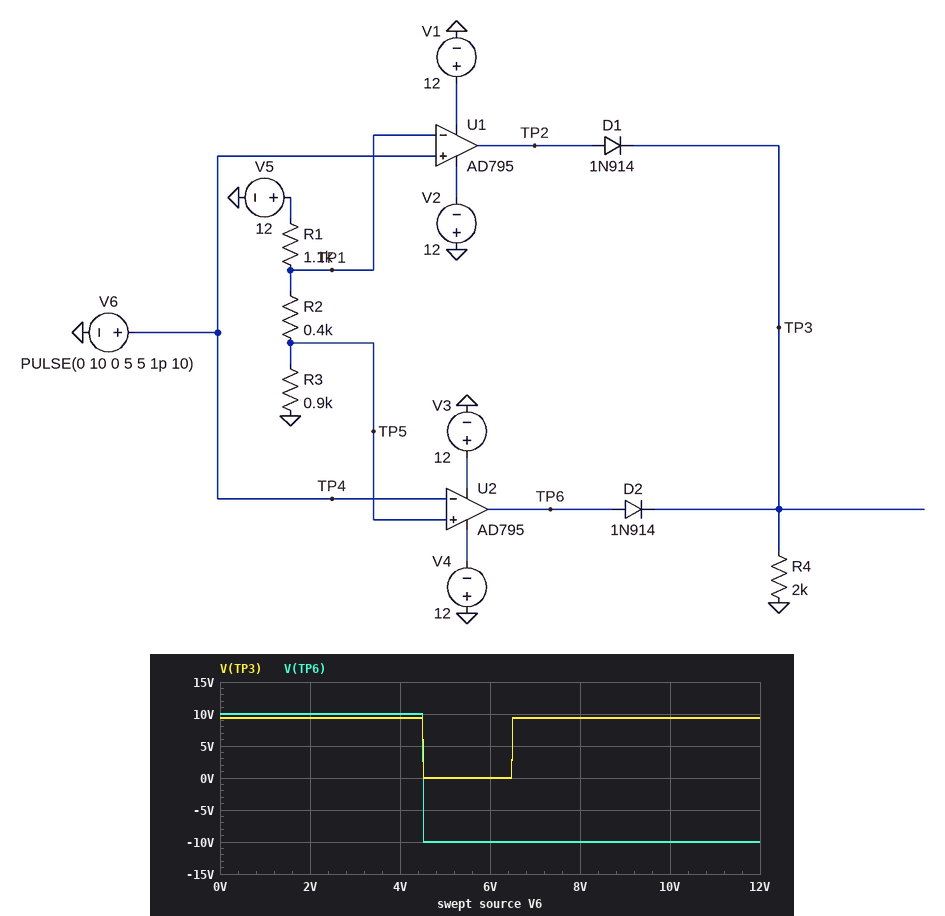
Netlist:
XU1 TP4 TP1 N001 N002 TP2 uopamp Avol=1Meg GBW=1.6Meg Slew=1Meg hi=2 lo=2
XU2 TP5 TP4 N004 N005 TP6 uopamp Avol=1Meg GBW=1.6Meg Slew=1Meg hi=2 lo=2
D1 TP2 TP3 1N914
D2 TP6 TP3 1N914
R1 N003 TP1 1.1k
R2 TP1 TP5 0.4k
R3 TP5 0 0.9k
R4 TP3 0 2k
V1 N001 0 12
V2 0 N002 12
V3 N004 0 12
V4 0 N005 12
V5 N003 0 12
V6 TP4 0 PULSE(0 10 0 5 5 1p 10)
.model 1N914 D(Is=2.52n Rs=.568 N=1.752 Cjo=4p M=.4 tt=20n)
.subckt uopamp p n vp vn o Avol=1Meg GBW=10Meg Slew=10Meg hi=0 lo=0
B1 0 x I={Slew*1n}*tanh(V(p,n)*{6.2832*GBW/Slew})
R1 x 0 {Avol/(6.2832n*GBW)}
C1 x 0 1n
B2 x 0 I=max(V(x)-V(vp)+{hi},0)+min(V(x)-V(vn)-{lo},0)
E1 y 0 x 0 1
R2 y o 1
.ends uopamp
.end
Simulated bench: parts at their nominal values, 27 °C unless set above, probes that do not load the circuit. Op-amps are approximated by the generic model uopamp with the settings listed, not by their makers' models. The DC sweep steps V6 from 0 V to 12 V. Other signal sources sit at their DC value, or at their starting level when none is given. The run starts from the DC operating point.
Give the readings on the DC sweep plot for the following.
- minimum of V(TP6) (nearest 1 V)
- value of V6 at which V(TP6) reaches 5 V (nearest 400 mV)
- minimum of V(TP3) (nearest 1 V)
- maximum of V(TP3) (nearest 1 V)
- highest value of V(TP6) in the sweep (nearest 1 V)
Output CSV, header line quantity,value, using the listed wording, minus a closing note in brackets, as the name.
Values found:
quantity,value
minimum of V(TP6),-10 V
value of V6 at which V(TP6) reaches 5 V,4.4 V
minimum of V(TP3),0 V
maximum of V(TP3),9 V
highest value of V(TP6) in the sweep,10 V
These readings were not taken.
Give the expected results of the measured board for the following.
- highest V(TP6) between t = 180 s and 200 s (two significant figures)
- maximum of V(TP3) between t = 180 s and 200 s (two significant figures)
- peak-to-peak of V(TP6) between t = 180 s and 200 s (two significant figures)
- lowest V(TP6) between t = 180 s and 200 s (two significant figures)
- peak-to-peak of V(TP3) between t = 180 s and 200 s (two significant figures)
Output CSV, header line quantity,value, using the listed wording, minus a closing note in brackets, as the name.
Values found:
quantity,value
highest V(TP6) between t = 180 s and 200 s,10 V
maximum of V(TP3) between t = 180 s and 200 s,9.3 V
peak-to-peak of V(TP6) between t = 180 s and 200 s,20 V
lowest V(TP6) between t = 180 s and 200 s,-10 V
peak-to-peak of V(TP3) between t = 180 s and 200 s,9.3 V
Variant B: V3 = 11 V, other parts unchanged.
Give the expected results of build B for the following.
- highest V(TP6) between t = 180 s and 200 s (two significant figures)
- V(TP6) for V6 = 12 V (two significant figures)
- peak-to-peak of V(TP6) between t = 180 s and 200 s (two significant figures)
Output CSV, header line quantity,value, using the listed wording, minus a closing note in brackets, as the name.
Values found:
quantity,value
highest V(TP6) between t = 180 s and 200 s,9.0 V
V(TP6) for V6 = 12 V,-10 V
peak-to-peak of V(TP6) between t = 180 s and 200 s,19 V
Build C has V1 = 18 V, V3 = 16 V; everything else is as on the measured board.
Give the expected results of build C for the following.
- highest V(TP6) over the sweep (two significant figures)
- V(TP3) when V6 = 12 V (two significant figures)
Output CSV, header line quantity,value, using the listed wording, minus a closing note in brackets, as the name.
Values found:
quantity,value
highest V(TP6) over the sweep,14 V
V(TP3) when V6 = 12 V,15 V
